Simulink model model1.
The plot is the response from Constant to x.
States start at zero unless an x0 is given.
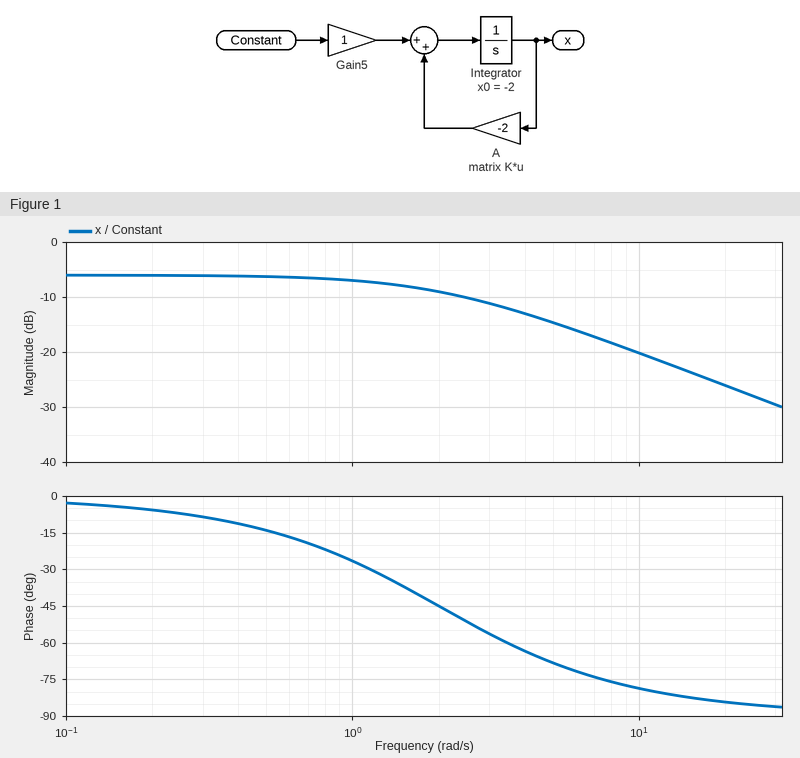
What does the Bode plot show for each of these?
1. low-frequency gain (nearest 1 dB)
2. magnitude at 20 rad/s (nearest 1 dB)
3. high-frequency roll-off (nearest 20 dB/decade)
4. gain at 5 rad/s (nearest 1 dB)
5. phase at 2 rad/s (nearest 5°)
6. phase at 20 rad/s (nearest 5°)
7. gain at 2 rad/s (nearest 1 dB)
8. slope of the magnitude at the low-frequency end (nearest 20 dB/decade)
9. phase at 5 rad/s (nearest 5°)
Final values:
-6 dB
-26 dB
-20 dB/decade
-15 dB
-45°
-85°
-9 dB
0 dB/decade
-70°
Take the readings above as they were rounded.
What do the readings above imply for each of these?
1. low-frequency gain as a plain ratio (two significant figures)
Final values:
0.50
